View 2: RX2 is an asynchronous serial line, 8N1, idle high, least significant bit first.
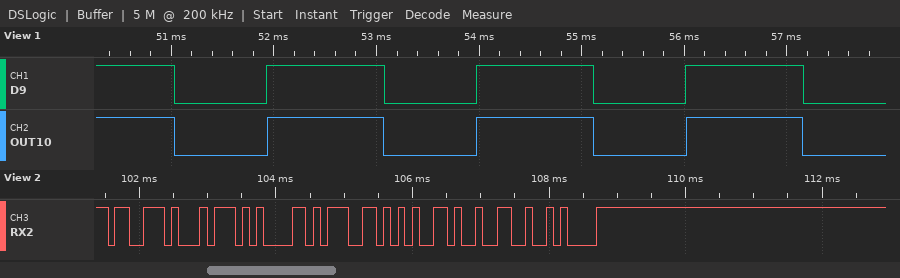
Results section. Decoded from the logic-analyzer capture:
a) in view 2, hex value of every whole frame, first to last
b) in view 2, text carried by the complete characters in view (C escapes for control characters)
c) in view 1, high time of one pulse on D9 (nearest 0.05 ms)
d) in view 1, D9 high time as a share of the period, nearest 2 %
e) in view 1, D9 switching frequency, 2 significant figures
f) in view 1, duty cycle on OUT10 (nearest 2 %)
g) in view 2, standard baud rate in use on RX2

73 74 61 67 65 32 0A
"stage2\n"
1.15 ms
56 %
490 Hz
56 %
9600 baud
